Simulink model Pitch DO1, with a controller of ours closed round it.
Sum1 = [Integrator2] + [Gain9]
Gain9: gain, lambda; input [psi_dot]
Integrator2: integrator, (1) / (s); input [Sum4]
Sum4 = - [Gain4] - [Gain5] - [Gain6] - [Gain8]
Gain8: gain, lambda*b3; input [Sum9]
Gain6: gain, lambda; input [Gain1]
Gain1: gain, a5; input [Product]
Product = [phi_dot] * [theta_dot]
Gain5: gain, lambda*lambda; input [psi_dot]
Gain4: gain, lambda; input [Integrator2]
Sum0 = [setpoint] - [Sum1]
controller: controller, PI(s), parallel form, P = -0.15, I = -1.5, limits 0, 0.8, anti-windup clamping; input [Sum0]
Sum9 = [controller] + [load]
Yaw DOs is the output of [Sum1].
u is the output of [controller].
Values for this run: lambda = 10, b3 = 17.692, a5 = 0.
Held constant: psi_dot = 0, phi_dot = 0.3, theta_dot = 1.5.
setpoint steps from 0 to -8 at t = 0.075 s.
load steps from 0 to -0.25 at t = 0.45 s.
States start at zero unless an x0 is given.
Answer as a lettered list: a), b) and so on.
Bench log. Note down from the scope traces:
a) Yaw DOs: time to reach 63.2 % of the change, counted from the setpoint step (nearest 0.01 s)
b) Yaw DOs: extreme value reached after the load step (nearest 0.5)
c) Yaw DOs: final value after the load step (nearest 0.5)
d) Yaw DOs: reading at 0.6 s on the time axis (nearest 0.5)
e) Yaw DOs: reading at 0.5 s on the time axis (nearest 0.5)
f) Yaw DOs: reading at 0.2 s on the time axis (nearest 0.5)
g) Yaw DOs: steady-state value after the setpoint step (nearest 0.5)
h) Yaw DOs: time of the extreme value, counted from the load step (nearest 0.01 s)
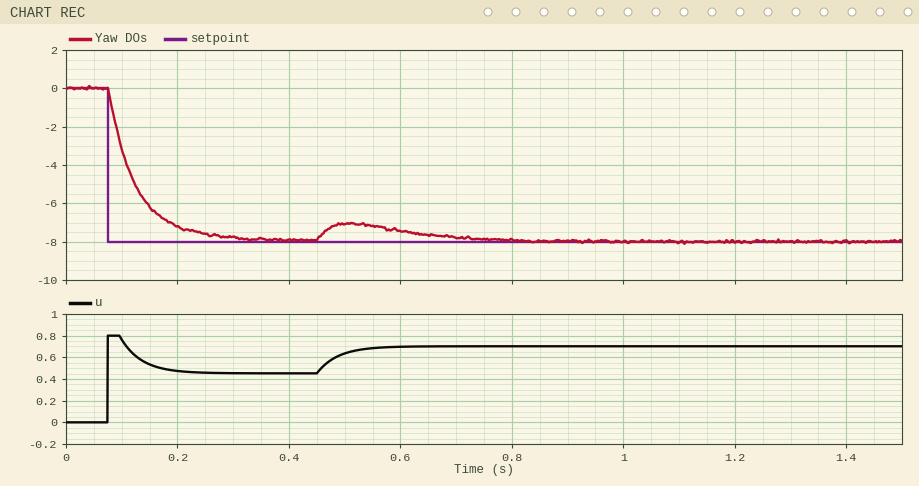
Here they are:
a) 0.05 s
b) -7.0
c) -8.0
d) -7.5
e) -7.0
f) -7.0
g) -8.0
h) 0.06 s
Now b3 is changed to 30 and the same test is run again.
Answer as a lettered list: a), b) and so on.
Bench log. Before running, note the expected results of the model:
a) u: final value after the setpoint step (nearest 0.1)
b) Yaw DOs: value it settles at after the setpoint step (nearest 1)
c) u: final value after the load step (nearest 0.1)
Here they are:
a) 0.3
b) -8
c) 0.5
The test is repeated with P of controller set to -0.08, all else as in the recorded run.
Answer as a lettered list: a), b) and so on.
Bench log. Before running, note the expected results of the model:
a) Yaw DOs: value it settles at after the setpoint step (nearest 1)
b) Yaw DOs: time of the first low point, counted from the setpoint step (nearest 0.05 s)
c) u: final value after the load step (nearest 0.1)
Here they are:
a) -8
b) 0.20 s
c) 0.7
